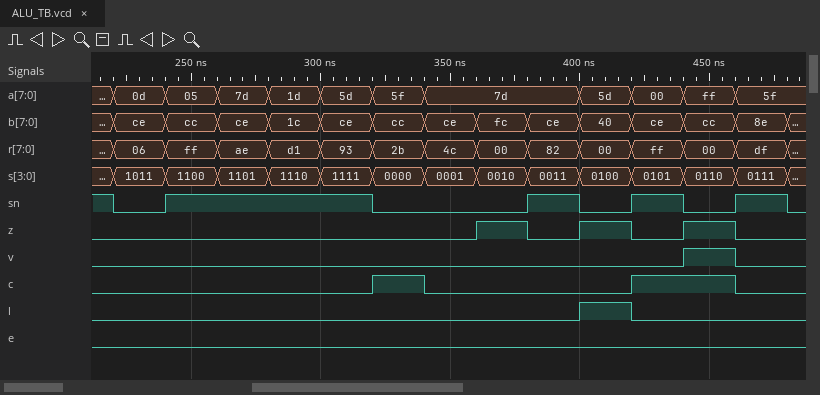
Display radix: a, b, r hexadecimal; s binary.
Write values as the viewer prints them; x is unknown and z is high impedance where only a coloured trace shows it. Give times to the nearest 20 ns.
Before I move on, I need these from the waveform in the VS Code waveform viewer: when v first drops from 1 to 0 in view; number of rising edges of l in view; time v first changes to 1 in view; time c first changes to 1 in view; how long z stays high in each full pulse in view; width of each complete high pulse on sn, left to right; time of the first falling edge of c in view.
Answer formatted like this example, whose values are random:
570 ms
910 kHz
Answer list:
460 ns
1
440 ns
320 ns
20 ns, 20 ns, 20 ns
80 ns, 20 ns, 20 ns, 20 ns
340 ns
